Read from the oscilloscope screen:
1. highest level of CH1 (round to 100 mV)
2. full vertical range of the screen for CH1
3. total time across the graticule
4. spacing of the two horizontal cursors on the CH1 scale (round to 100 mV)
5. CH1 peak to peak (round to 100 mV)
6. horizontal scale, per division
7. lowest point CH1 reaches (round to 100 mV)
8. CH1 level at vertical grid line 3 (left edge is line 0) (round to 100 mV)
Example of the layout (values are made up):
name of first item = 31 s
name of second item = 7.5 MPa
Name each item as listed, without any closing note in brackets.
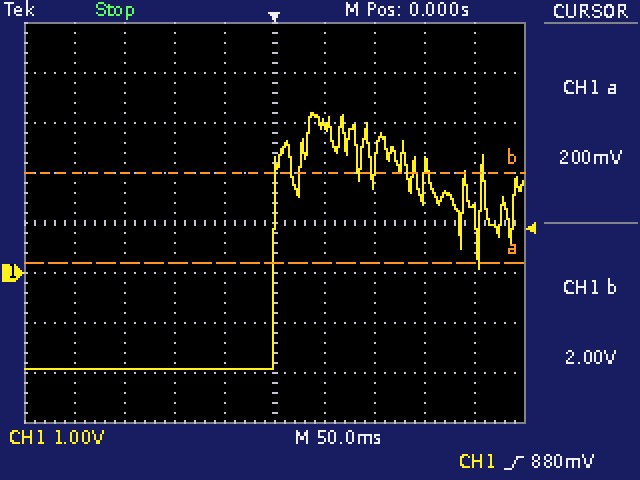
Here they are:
highest level of CH1 = 3.2 V
full vertical range of the screen for CH1 = 8 V
total time across the graticule = 500 ms
spacing of the two horizontal cursors on the CH1 scale = 1.8 V
CH1 peak to peak = 5.1 V
horizontal scale, per division = 50 ms
lowest point CH1 reaches = -1.9 V
CH1 level at vertical grid line 3 (left edge is line 0) = -1.9 V
